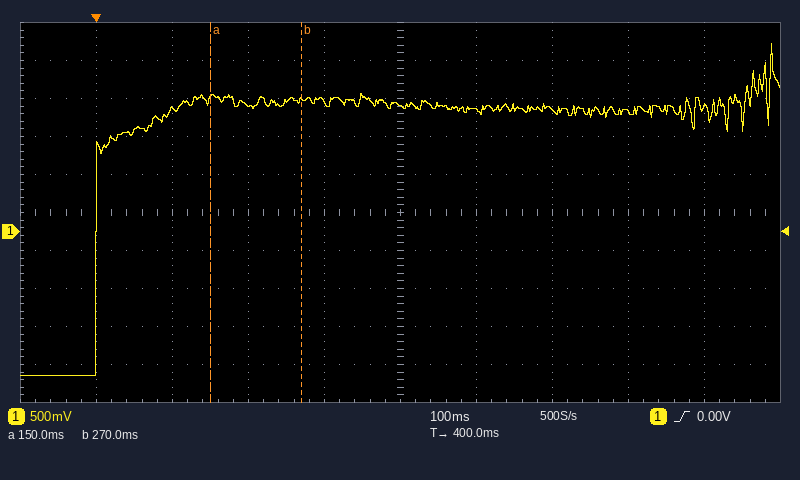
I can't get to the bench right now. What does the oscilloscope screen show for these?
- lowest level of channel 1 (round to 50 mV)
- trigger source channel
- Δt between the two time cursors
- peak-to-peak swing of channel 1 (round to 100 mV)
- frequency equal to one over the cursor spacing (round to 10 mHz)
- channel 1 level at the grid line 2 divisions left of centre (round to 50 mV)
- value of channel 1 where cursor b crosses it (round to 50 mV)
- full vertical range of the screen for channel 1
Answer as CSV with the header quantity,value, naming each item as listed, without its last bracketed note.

quantity,value
lowest level of channel 1,-1.90 V
trigger source channel,channel 1
Δt between the two time cursors,120 ms
peak-to-peak swing of channel 1,4.40 V
frequency equal to one over the cursor spacing,8.33 Hz
channel 1 level at the grid line 2 divisions left of centre,1.65 V
value of channel 1 where cursor b crosses it,1.70 V
full vertical range of the screen for channel 1,5 V
